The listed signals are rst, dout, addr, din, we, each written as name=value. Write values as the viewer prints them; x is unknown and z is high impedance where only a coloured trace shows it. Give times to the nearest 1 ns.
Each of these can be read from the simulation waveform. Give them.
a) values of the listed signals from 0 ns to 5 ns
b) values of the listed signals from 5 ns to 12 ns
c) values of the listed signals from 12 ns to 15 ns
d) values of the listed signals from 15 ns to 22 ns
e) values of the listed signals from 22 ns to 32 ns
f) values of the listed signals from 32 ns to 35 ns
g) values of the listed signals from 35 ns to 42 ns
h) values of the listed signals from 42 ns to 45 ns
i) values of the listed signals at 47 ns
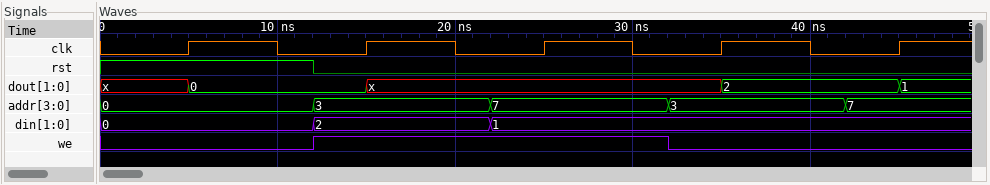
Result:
rst=1, dout=x, addr=0, din=0, we=0
rst=1, dout=0, addr=0, din=0, we=0
rst=0, dout=0, addr=3, din=2, we=1
rst=0, dout=x, addr=3, din=2, we=1
rst=0, dout=x, addr=7, din=1, we=1
rst=0, dout=x, addr=3, din=1, we=0
rst=0, dout=2, addr=3, din=1, we=0
rst=0, dout=2, addr=7, din=1, we=0
rst=0, dout=1, addr=7, din=1, we=0
